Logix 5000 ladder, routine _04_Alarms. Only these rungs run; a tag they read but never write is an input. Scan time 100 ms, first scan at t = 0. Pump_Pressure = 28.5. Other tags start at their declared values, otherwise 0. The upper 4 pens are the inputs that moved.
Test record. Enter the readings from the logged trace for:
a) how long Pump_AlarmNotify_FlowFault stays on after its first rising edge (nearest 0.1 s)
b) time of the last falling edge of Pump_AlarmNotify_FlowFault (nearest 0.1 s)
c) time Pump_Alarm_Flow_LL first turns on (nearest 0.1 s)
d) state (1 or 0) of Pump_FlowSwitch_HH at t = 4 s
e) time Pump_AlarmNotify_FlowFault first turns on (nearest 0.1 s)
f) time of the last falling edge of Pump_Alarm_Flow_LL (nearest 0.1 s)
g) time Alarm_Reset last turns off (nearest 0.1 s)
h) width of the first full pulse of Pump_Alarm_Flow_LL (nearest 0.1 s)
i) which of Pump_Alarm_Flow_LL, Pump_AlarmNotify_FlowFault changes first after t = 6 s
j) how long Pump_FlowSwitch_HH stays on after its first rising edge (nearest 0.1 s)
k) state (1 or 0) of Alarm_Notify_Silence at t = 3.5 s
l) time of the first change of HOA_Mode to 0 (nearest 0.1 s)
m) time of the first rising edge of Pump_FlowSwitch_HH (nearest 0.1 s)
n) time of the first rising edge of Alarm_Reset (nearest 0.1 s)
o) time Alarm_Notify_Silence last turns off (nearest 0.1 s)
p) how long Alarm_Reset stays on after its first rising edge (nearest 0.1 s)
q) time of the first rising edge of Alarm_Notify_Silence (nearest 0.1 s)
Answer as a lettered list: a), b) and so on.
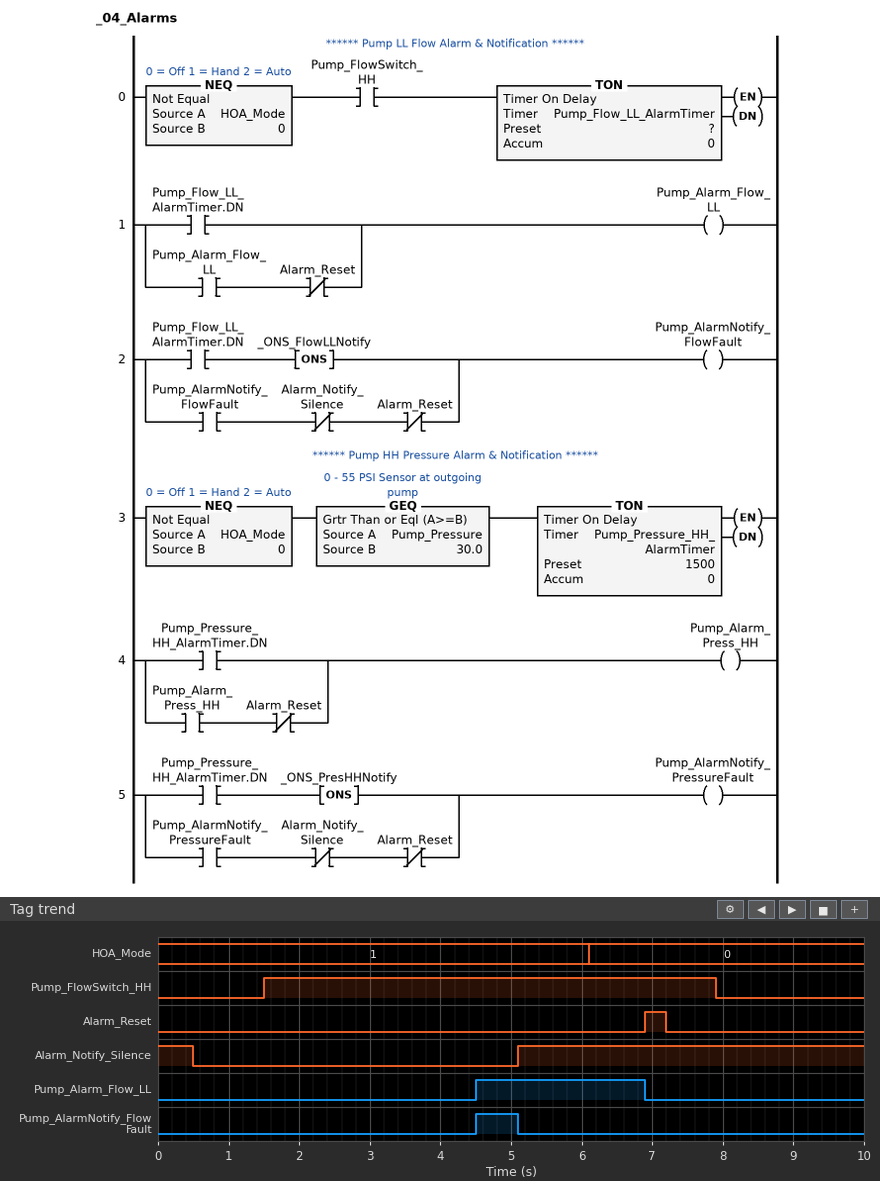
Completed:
a) 0.6 s
b) 5.1 s
c) 4.5 s
d) 1
e) 4.5 s
f) 6.9 s
g) 7.2 s
h) 2.4 s
i) Pump_Alarm_Flow_LL
j) 6.4 s
k) 0
l) 6.1 s
m) 1.5 s
n) 6.9 s
o) 0.5 s
p) 0.3 s
q) 5.1 s
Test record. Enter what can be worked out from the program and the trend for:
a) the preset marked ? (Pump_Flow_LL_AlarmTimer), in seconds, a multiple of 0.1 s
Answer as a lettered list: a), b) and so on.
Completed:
a) 3.0 s
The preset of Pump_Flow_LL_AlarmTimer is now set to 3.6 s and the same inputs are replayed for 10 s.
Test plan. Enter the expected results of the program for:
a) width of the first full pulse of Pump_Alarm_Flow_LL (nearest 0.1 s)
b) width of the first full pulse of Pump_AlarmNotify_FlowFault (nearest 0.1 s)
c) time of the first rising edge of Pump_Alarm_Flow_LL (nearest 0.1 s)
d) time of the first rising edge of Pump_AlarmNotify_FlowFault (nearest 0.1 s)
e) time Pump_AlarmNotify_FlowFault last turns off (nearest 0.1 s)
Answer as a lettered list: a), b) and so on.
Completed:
a) 1.8 s
b) 0.1 s
c) 5.1 s
d) 5.1 s
e) 5.2 s
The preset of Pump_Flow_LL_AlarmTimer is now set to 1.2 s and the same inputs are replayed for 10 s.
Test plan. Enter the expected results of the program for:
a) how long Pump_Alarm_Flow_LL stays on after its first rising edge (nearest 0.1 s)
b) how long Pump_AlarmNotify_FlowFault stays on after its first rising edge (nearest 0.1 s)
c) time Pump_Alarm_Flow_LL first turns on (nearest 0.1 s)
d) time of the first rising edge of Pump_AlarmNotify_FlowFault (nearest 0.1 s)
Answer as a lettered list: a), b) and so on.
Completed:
a) 4.2 s
b) 2.4 s
c) 2.7 s
d) 2.7 s
